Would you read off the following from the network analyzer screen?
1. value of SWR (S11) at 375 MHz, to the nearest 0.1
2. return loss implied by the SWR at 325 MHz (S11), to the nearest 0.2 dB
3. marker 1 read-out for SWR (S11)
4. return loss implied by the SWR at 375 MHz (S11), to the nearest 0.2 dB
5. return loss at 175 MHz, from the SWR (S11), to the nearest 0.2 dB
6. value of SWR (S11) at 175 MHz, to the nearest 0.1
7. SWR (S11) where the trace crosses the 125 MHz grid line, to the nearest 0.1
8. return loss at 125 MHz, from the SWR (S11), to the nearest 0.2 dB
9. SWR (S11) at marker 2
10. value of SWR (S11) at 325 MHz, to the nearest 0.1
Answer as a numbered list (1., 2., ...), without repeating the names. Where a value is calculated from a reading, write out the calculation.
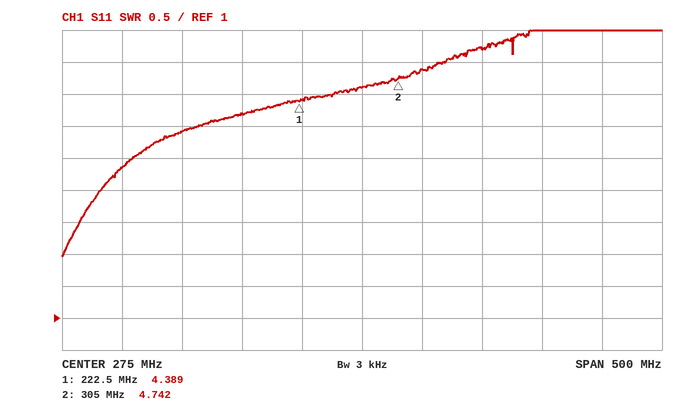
1. 5.2
2. −20 log10((4.9 − 1)/(4.9 + 1)) ≈ 3.6 dB
3. 4.389
4. −20 log10((5.2 − 1)/(5.2 + 1)) ≈ 3.4 dB
5. −20 log10((4.2 − 1)/(4.2 + 1)) ≈ 4.2 dB
6. 4.2
7. 3.9
8. −20 log10((3.9 − 1)/(3.9 + 1)) ≈ 4.6 dB
9. 4.742
10. 4.9
